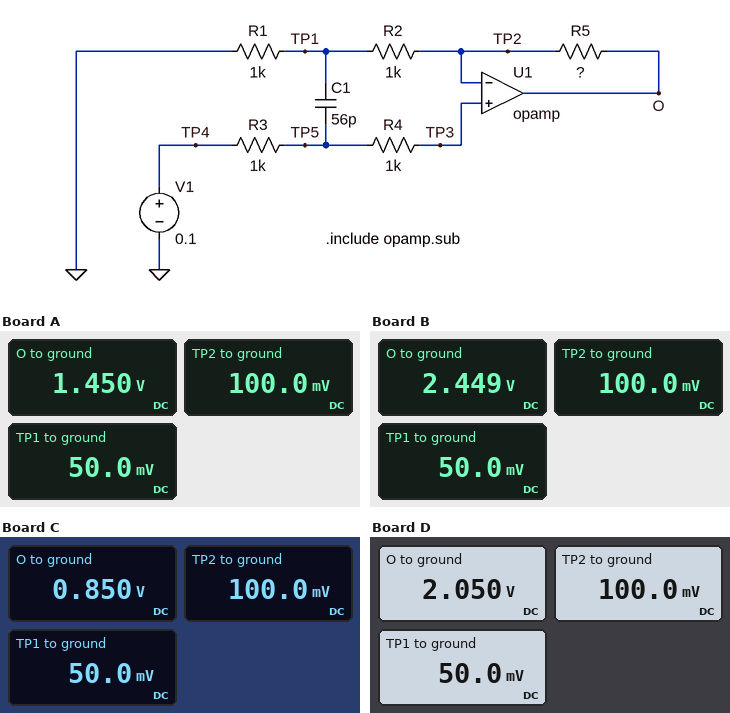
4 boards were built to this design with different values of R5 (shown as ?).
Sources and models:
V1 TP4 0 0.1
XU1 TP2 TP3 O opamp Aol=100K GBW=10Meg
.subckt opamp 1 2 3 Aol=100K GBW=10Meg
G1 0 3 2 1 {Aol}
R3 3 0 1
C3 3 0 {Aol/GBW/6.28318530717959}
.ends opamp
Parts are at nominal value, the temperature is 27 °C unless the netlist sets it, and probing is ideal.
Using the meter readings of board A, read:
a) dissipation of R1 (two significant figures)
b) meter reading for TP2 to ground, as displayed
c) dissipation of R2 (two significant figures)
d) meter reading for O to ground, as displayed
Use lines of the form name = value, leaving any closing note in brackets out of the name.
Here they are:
dissipation of R1 = 2.5 µW
meter reading for TP2 to ground, as displayed = 100.0 mV
dissipation of R2 = 2.5 µW
meter reading for O to ground, as displayed = 1.450 V
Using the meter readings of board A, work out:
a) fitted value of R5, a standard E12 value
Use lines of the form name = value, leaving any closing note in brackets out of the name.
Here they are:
fitted value of R5, a standard E12 value = 27 kΩ
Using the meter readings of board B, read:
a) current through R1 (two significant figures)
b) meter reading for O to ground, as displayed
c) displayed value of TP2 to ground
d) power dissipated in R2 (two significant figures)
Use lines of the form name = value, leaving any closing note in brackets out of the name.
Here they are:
current through R1 = 50 µA
meter reading for O to ground, as displayed = 2.449 V
displayed value of TP2 to ground = 100.0 mV
power dissipated in R2 = 2.5 µW
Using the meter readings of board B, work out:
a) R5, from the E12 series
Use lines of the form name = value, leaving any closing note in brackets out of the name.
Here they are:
R5, from the E12 series = 47 kΩ
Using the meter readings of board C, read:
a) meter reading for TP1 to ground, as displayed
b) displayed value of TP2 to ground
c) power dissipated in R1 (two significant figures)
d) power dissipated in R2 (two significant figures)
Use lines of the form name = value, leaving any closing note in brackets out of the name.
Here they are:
meter reading for TP1 to ground, as displayed = 50.0 mV
displayed value of TP2 to ground = 100.0 mV
power dissipated in R1 = 2.5 µW
power dissipated in R2 = 2.5 µW
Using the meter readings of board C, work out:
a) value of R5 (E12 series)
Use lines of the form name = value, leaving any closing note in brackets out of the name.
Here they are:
value of R5 = 15 kΩ
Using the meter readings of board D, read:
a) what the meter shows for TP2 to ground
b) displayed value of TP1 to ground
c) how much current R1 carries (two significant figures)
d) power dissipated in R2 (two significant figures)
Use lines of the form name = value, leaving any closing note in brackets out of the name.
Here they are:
what the meter shows for TP2 to ground = 100.0 mV
displayed value of TP1 to ground = 50.0 mV
how much current R1 carries = 50 µA
power dissipated in R2 = 2.5 µW
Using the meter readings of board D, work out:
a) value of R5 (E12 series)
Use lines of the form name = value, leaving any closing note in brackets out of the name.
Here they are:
value of R5 = 39 kΩ
